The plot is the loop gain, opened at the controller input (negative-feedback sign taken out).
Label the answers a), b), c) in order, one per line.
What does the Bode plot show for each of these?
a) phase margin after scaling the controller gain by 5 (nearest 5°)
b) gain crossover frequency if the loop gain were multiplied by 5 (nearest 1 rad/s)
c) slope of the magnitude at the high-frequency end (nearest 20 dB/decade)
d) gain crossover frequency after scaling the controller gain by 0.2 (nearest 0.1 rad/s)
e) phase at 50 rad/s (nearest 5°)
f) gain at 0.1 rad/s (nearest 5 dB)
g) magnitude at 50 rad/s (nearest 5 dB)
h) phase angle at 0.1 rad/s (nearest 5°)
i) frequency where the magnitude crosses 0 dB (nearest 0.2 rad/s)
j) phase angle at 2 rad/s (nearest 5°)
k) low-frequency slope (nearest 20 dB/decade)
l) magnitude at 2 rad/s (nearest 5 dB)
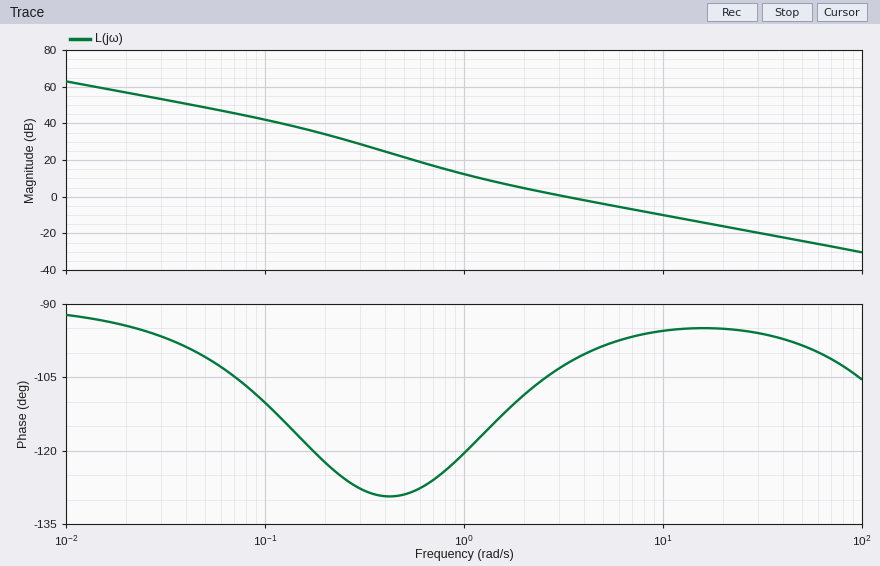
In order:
a) 85°
b) 16 rad/s
c) -20 dB/decade
d) 0.9 rad/s
e) -100°
f) 40 dB
g) -25 dB
h) -110°
i) 3.2 rad/s
j) -110°
k) -20 dB/decade
l) 5 dB
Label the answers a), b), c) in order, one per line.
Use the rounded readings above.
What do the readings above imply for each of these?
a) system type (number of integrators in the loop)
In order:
a) 1
